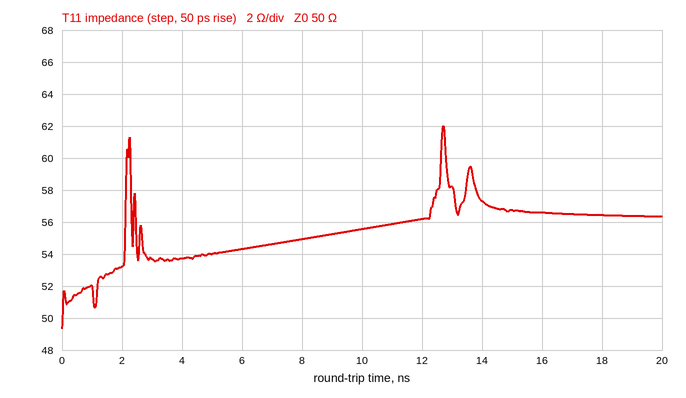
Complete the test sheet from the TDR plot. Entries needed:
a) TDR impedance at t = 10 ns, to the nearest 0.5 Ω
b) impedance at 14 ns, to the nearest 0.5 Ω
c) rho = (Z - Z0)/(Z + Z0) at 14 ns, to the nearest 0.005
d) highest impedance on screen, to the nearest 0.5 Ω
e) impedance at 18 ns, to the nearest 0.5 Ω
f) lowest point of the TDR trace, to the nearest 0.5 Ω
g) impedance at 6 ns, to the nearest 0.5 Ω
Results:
55.5 Ω
57.5 Ω
+0.070
62.0 Ω
56.5 Ω
49.5 Ω
54.5 Ω
